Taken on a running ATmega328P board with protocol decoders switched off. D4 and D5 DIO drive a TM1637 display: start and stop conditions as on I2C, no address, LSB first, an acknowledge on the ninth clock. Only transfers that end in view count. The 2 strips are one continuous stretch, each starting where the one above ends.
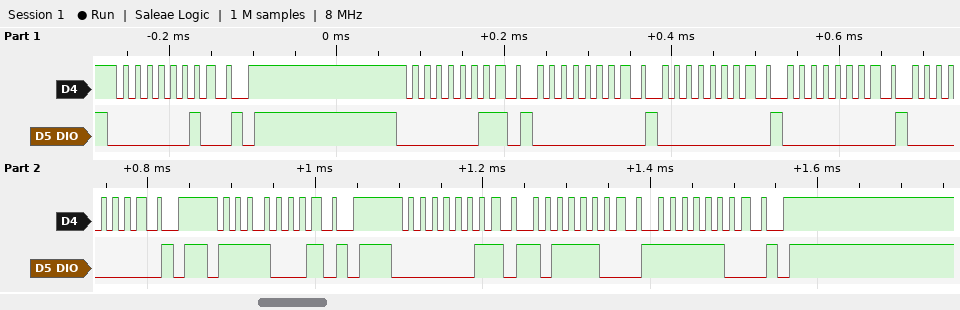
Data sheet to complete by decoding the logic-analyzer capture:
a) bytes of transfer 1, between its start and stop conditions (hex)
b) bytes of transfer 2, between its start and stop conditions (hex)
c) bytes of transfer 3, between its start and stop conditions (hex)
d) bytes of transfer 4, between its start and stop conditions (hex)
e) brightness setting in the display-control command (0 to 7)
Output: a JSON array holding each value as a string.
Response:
["40", "C0 00 00 00 00", "8F", "C0 3D 3F", "7"]
